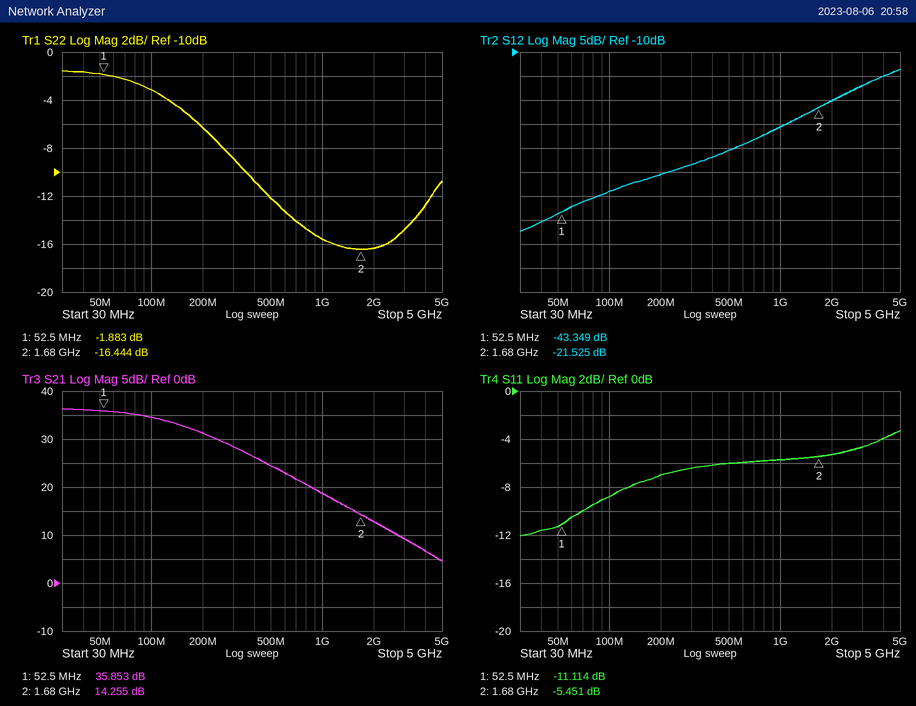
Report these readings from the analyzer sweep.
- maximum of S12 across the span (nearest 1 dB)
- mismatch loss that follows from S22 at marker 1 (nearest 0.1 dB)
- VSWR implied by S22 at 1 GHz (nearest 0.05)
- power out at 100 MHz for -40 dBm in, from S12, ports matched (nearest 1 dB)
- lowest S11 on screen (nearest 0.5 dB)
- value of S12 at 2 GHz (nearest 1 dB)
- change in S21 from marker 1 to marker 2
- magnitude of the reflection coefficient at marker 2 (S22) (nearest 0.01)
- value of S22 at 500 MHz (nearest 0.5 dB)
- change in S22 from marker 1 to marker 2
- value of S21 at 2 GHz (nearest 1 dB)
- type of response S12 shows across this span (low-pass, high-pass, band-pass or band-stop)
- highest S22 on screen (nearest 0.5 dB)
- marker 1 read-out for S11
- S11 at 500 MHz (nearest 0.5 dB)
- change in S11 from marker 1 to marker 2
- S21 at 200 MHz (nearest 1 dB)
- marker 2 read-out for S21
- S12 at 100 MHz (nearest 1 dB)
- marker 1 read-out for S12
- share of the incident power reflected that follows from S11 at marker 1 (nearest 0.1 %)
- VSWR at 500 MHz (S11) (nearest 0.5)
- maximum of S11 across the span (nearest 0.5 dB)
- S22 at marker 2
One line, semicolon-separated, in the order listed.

-14 dB; 4.5 dB; 1.40; -79 dBm; -12.0 dB; -20 dB; -21.598 dB; 0.15; -12.0 dB; -14.561 dB; 13 dB; high-pass; -1.5 dB; -11.114 dB; -6.0 dB; 5.663 dB; 31 dB; 14.255 dB; -39 dB; -43.349 dB; 7.7 %; 3.0; -3.5 dB; -16.444 dB
